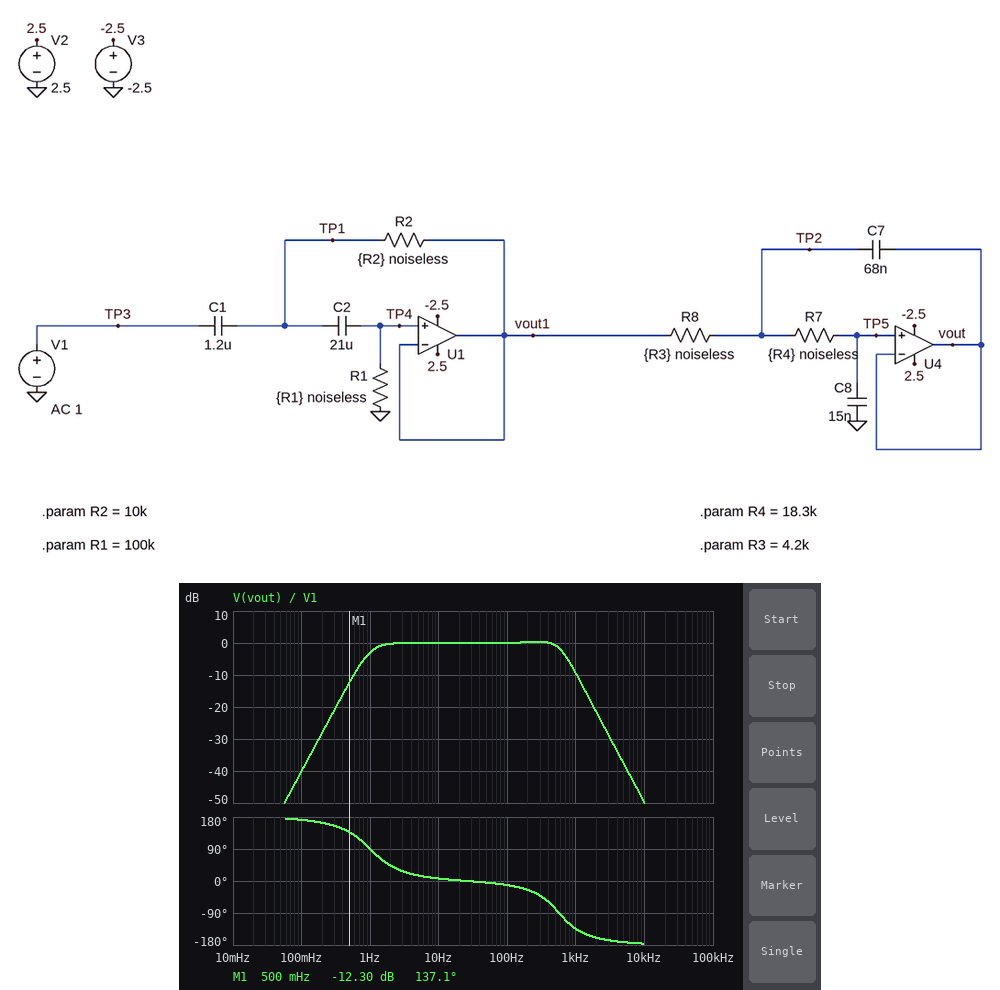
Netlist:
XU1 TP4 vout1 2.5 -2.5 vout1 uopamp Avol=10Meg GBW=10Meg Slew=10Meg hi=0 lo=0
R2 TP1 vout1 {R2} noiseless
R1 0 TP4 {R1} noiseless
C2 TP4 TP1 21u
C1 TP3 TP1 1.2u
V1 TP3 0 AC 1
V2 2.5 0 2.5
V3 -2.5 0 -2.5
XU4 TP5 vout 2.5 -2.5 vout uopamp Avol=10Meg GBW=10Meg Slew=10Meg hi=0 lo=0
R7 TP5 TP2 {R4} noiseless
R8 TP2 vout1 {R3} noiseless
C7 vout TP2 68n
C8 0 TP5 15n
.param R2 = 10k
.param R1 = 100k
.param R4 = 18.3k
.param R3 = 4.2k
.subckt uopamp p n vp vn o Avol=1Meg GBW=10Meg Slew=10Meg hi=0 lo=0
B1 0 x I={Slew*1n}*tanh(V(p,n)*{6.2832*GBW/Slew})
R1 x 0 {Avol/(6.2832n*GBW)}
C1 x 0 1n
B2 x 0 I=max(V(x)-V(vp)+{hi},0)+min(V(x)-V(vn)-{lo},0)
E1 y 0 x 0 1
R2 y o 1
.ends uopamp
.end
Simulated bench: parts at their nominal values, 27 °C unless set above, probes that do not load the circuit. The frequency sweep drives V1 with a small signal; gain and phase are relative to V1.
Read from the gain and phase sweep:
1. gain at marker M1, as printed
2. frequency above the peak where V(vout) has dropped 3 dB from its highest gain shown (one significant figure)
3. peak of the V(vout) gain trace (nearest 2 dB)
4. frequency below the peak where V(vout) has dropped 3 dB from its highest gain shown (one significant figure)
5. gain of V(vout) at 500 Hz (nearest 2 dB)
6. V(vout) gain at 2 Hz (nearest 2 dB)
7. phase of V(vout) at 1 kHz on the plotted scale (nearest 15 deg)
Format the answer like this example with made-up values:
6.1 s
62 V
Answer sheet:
-12.30 dB
600 Hz
0 dB
1 Hz
0 dB
0 dB
-135 deg
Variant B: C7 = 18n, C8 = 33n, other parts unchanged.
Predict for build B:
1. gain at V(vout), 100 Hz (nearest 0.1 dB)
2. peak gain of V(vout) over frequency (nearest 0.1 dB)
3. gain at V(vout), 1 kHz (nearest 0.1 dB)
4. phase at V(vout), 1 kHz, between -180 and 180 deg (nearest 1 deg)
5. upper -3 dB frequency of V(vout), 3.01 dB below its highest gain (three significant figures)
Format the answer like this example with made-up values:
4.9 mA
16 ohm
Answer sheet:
-0.7 dB
0 dB
-13.5 dB
-100 deg
234 Hz
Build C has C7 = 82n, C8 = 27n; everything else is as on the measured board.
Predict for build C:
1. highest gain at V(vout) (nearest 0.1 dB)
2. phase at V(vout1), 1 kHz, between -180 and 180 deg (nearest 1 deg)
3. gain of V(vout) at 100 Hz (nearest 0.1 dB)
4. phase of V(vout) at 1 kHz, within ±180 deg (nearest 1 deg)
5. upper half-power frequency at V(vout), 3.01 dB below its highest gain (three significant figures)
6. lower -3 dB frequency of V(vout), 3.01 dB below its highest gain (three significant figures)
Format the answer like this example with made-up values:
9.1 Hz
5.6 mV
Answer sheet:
0 dB
0 deg
-0.1 dB
-146 deg
370 Hz
992 mHz
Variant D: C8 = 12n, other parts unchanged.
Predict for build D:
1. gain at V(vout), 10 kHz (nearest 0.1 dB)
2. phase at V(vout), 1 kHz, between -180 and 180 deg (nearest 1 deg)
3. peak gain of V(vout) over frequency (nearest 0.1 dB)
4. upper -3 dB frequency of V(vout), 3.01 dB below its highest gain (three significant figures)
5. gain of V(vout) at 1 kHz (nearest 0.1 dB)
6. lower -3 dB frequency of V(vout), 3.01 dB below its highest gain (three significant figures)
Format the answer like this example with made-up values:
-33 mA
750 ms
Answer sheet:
-47.9 dB
-131 deg
0.8 dB
732 Hz
-7.0 dB
1.10 Hz
